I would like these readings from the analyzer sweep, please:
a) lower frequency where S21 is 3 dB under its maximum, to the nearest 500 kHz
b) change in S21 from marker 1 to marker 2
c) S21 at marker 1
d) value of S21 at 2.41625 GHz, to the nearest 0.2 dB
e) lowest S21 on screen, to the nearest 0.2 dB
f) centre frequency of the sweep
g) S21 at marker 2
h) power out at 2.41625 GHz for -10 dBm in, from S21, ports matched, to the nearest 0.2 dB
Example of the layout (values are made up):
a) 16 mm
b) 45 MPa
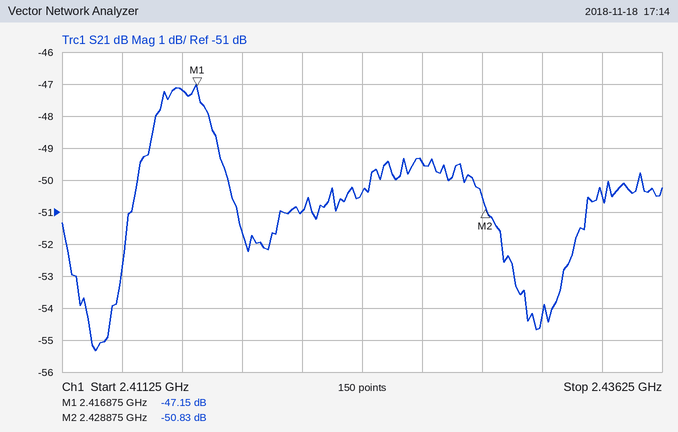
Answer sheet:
a) 2.4145 GHz
b) -3.68 dB
c) -47.15 dB
d) -47.2 dB
e) -55.4 dB
f) 2.42375 GHz
g) -50.83 dB
h) -57.2 dBm
